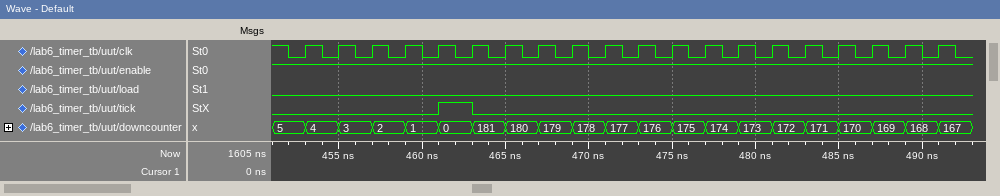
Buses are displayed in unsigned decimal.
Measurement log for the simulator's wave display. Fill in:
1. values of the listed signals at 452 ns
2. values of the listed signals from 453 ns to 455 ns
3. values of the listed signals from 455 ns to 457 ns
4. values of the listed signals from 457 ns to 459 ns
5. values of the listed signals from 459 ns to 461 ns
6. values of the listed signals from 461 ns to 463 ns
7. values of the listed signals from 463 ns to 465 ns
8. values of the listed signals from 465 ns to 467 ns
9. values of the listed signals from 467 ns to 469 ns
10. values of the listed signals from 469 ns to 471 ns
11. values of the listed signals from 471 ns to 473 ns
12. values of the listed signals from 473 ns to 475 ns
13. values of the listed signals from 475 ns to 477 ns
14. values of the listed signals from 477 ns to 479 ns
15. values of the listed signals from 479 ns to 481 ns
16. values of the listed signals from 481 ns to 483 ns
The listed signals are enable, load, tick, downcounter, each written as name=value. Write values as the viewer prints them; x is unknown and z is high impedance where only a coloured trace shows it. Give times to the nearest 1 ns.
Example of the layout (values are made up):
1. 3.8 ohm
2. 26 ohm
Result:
1. enable=1, load=0, tick=0, downcounter=5
2. enable=1, load=0, tick=0, downcounter=4
3. enable=1, load=0, tick=0, downcounter=3
4. enable=1, load=0, tick=0, downcounter=2
5. enable=1, load=0, tick=0, downcounter=1
6. enable=1, load=0, tick=1, downcounter=0
7. enable=1, load=0, tick=0, downcounter=181
8. enable=1, load=0, tick=0, downcounter=180
9. enable=1, load=0, tick=0, downcounter=179
10. enable=1, load=0, tick=0, downcounter=178
11. enable=1, load=0, tick=0, downcounter=177
12. enable=1, load=0, tick=0, downcounter=176
13. enable=1, load=0, tick=0, downcounter=175
14. enable=1, load=0, tick=0, downcounter=174
15. enable=1, load=0, tick=0, downcounter=173
16. enable=1, load=0, tick=0, downcounter=172
